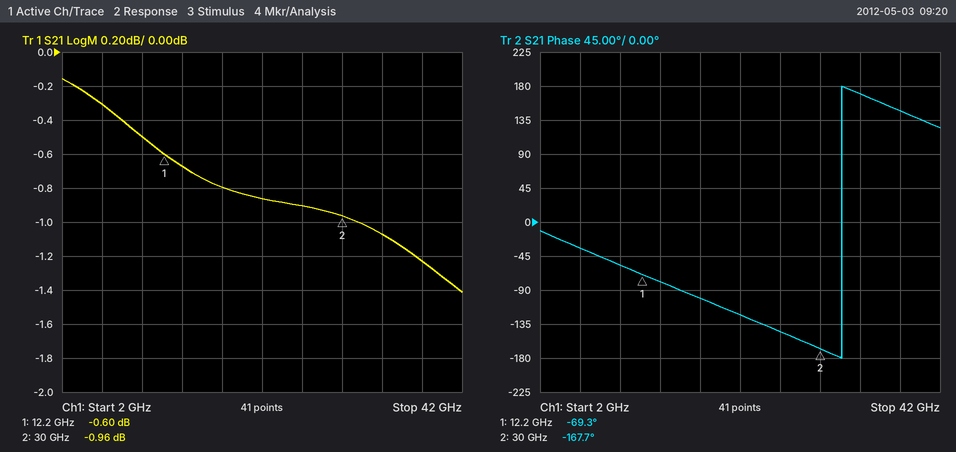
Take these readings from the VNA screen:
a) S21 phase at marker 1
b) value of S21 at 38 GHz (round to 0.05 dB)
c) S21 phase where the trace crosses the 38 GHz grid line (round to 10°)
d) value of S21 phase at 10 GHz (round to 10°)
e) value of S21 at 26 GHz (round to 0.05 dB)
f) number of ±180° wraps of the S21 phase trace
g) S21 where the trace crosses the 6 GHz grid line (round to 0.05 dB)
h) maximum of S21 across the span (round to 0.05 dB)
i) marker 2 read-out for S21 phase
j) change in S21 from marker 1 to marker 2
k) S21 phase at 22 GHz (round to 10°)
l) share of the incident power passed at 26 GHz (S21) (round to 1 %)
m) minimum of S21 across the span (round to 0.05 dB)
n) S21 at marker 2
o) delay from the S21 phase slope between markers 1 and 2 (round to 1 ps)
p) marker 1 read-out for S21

-69.3°
-1.25 dB
150°
-60°
-0.90 dB
1
-0.30 dB
-0.15 dB
-167.7°
-0.36 dB
-120°
81 %
-1.40 dB
-0.96 dB
15 ps
-0.60 dB
